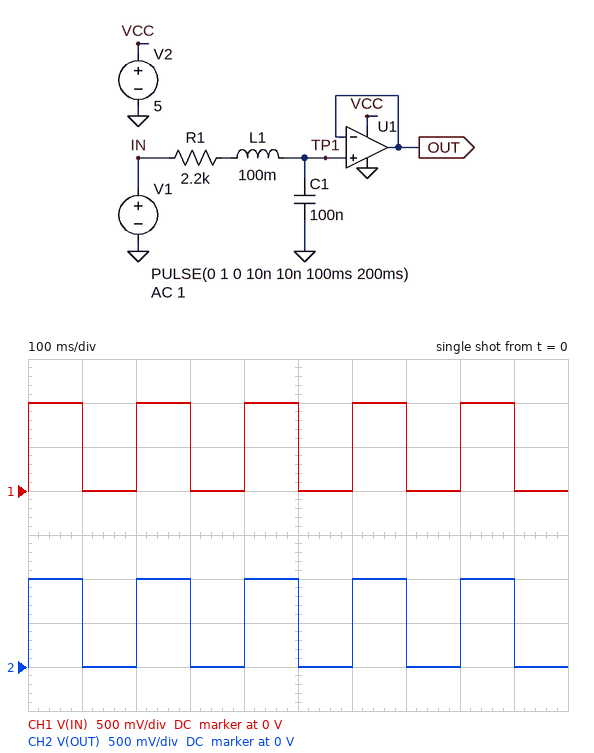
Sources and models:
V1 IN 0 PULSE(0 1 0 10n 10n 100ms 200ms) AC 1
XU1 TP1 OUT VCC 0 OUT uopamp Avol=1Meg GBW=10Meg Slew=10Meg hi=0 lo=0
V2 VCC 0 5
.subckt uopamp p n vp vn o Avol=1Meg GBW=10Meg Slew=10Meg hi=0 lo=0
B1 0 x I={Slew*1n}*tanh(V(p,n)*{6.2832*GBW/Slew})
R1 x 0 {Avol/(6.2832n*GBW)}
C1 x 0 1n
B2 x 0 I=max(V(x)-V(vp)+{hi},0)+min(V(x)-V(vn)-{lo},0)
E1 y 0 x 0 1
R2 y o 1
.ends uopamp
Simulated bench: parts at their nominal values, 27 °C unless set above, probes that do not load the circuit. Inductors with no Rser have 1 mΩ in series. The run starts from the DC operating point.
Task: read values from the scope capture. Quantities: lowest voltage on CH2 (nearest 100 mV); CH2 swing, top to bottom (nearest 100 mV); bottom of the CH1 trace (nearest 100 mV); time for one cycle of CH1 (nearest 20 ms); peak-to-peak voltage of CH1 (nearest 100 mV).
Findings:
0 V
1.0 V
0 V
200 ms
1.0 V
